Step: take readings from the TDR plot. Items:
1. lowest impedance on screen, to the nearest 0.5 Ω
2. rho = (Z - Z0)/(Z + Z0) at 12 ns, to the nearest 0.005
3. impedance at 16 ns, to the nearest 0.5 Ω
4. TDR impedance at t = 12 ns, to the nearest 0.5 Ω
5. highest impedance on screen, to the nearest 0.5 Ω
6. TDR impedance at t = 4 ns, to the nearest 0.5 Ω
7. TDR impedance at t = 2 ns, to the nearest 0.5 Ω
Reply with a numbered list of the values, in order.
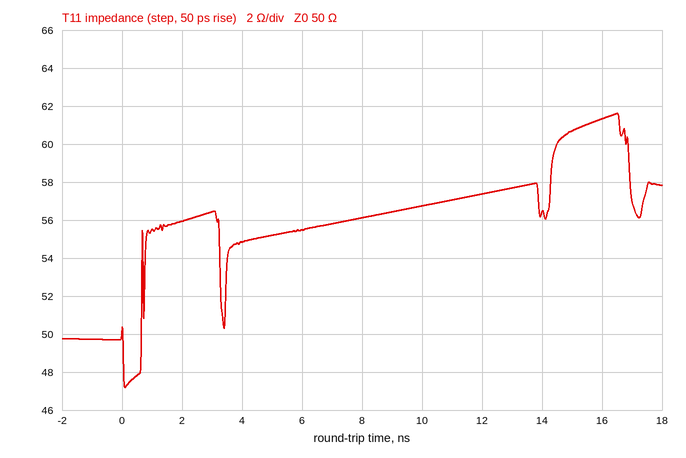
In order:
1. 47.0 Ω
2. +0.070
3. 61.5 Ω
4. 57.5 Ω
5. 61.5 Ω
6. 55.0 Ω
7. 56.0 Ω
